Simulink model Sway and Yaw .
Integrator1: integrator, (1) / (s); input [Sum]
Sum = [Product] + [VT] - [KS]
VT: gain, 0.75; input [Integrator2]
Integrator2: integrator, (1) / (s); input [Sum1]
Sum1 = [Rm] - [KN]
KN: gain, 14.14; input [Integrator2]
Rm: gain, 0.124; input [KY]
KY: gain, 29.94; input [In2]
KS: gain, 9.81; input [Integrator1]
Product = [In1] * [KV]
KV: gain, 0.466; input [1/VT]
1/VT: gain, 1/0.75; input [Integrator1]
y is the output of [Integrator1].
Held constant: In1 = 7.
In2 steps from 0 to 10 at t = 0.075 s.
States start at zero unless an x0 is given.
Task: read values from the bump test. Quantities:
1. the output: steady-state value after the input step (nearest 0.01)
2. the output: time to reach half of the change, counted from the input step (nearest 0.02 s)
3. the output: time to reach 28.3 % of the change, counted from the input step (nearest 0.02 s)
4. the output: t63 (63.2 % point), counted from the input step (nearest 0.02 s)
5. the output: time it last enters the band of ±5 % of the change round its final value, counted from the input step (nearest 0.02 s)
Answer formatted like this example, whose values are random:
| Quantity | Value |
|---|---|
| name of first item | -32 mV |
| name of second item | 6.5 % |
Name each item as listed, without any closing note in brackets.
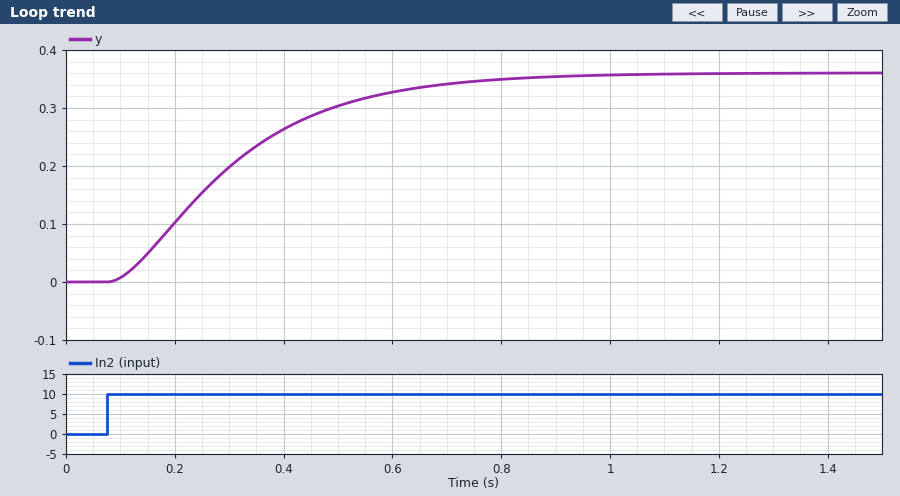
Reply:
| Quantity | Value |
|---|---|
| the output: steady-state value after the input step | 0.36 |
| the output: time to reach half of the change, counted from the input step | 0.20 s |
| the output: time to reach 28.3 % of the change, counted from the input step | 0.12 s |
| the output: t63 (63.2 % point), counted from the input step | 0.26 s |
| the output: time it last enters the band of ±5 % of the change round its final value, counted from the input step | 0.64 s |
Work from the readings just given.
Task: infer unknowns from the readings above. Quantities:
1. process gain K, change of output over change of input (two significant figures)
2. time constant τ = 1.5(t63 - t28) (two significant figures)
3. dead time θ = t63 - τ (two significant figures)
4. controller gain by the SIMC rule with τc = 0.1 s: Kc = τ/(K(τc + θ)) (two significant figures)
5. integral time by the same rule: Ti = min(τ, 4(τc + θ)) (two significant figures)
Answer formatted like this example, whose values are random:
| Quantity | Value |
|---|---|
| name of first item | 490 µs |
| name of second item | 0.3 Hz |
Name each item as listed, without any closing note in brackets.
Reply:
| Quantity | Value |
|---|---|
| process gain K, change of output over change of input | 0.036 |
| time constant τ = 1.5(t63 - t28) | 0.21 s |
| dead time θ = t63 - τ | 0.050 s |
| controller gain by the SIMC rule with τc = 0.1 s: Kc = τ/(K(τc + θ)) | 39 |
| integral time by the same rule: Ti = min(τ, 4(τc + θ)) | 0.21 s |
